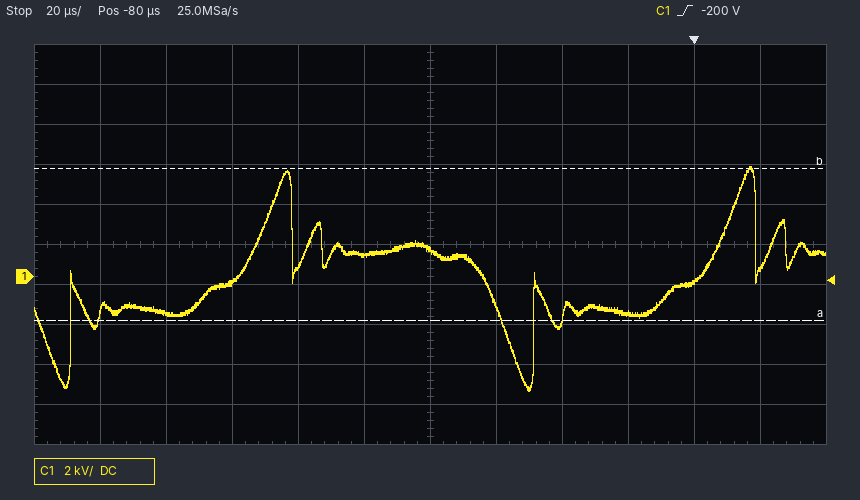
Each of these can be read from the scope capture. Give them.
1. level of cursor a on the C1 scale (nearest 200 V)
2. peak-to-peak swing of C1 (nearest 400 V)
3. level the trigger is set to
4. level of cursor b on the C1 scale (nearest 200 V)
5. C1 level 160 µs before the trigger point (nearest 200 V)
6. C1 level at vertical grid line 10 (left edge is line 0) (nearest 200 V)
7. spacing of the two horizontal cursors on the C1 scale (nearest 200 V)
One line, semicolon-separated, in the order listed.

-2.2 kV; 11.2 kV; -200 V; 5.4 kV; -1.8 kV; -200 V; 7.6 kV
